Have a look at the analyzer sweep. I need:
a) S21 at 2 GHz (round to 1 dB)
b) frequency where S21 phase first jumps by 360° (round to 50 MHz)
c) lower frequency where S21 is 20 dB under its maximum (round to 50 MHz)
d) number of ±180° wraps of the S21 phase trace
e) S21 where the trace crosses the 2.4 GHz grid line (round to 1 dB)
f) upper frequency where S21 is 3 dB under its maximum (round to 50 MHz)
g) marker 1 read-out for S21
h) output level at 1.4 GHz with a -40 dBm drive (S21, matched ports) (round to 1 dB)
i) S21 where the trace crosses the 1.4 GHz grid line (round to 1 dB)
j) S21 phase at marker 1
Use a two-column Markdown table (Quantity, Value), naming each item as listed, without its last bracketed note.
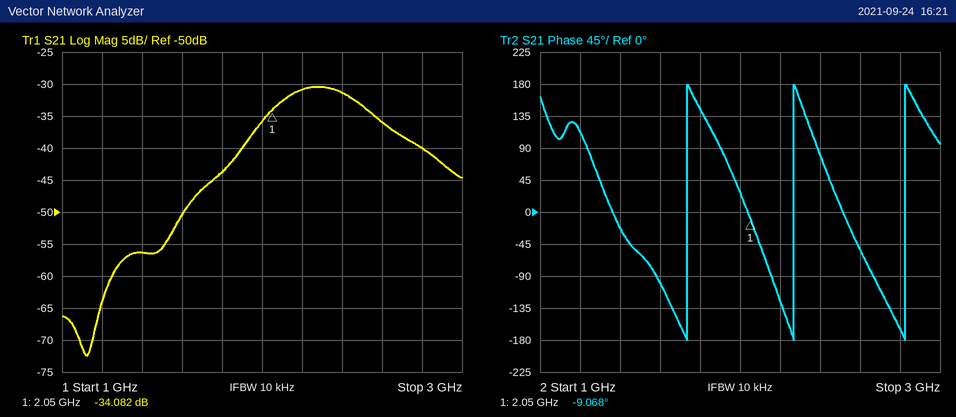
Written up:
| Quantity | Value |
|---|---|
| S21 at 2 GHz | -36 dB |
| frequency where S21 phase first jumps by 360° | 1.75 GHz |
| lower frequency where S21 is 20 dB under its maximum | 1.60 GHz |
| number of ±180° wraps of the S21 phase trace | 3 |
| S21 where the trace crosses the 2.4 GHz grid line | -31 dB |
| upper frequency where S21 is 3 dB under its maximum | 2.50 GHz |
| marker 1 read-out for S21 | -34.082 dB |
| output level at 1.4 GHz with a -40 dBm drive (S21, matched ports) | -96 dBm |
| S21 where the trace crosses the 1.4 GHz grid line | -56 dB |
| S21 phase at marker 1 | -9.068° |
